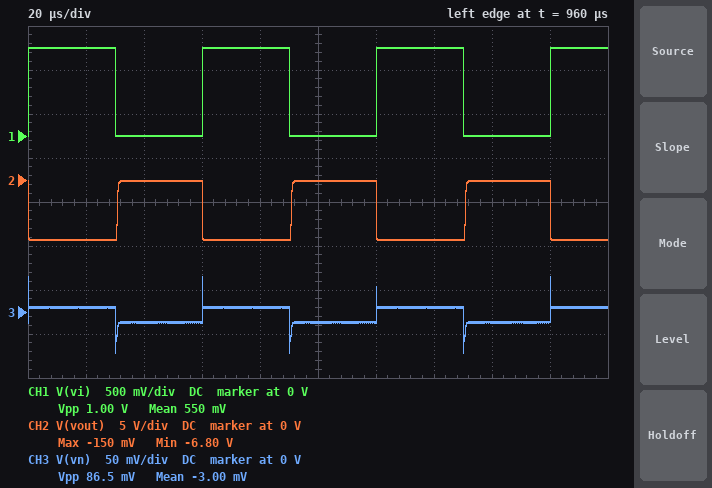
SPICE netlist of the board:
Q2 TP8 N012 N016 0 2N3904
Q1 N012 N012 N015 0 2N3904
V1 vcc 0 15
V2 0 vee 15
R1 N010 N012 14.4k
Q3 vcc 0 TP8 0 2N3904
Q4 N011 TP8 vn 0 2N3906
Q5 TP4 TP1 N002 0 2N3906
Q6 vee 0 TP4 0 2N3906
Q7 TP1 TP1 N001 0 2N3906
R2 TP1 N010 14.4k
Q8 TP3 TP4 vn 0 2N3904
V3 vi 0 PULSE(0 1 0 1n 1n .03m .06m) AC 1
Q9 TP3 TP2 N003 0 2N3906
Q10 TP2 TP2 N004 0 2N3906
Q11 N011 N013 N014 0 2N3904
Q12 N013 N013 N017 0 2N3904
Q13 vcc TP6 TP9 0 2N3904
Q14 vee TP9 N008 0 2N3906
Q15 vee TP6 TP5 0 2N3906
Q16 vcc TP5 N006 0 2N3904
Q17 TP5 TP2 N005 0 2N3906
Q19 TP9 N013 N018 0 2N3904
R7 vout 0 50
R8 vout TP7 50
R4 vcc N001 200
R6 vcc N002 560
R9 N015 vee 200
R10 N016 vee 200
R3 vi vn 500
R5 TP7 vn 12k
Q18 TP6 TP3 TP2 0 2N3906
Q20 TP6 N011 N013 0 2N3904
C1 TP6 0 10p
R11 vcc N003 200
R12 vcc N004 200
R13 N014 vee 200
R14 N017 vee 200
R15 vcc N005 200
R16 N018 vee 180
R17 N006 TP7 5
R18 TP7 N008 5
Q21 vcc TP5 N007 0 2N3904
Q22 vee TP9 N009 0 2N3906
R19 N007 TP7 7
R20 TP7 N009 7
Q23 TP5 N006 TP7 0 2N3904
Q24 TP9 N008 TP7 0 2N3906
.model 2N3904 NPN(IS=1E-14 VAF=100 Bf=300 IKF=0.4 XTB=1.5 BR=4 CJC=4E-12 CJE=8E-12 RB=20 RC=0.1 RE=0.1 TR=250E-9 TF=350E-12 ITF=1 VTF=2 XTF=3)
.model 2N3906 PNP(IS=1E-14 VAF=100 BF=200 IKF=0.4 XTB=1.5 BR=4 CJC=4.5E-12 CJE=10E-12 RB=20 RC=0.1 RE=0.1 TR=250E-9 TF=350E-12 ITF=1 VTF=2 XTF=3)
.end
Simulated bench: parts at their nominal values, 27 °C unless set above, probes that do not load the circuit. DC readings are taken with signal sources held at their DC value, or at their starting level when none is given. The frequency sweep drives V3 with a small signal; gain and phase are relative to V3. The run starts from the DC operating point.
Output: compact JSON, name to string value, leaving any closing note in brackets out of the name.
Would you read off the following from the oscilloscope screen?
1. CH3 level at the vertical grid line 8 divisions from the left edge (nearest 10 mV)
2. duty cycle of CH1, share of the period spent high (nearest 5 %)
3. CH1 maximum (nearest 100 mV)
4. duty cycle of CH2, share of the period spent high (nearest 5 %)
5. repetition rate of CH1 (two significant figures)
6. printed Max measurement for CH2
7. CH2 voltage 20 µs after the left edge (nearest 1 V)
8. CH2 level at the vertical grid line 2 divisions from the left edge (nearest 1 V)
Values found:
{"CH3 level at the vertical grid line 8 divisions from the left edge": "-10 mV", "duty cycle of CH1, share of the period spent high": "50 %", "CH1 maximum": "1.0 V", "duty cycle of CH2, share of the period spent high": "50 %", "repetition rate of CH1": "17 kHz", "printed Max measurement for CH2": "-150 mV", "CH2 voltage 20 µs after the left edge": "-7 V", "CH2 level at the vertical grid line 2 divisions from the left edge": "0 V"}
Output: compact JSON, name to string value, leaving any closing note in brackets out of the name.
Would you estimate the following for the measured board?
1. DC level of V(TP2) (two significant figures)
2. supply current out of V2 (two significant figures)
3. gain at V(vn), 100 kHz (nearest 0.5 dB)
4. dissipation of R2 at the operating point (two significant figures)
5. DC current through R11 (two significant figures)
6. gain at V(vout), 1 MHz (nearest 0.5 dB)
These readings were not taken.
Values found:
{"DC level of V(TP2)": "14 V", "supply current out of V2": "7.9 mA", "gain at V(vn), 100 kHz": "-45.0 dB", "dissipation of R2 at the operating point": "14 mW", "DC current through R11": "610 µA", "gain at V(vout), 1 MHz": "17.0 dB"}
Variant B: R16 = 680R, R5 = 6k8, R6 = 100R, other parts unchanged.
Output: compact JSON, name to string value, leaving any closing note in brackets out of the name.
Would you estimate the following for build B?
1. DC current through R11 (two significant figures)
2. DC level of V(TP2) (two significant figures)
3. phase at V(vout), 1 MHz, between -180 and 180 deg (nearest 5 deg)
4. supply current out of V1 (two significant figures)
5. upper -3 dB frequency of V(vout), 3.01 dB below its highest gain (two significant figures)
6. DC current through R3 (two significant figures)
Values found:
{"DC current through R11": "1.3 mA", "DC level of V(TP2)": "14 V", "phase at V(vout), 1 MHz, between -180 and 180 deg": "140 deg", "supply current out of V1": "11 mA", "upper -3 dB frequency of V(vout), 3.01 dB below its highest gain": "1.3 MHz", "DC current through R3": "16 µA"}
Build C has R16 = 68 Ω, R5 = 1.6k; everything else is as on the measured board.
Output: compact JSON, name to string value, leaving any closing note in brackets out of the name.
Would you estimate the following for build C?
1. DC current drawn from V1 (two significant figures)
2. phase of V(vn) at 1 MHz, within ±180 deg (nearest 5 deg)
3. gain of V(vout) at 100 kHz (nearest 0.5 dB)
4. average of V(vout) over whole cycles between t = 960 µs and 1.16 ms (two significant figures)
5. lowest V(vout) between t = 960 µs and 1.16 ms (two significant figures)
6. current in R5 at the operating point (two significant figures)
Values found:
{"DC current drawn from V1": "7.0 mA", "phase of V(vn) at 1 MHz, within ±180 deg": "80 deg", "gain of V(vout) at 100 kHz": "4.0 dB", "average of V(vout) over whole cycles between t = 960 µs and 1.16 ms": "-830 mV", "lowest V(vout) between t = 960 µs and 1.16 ms": "-1.6 V", "current in R5 at the operating point": "26 µA"}
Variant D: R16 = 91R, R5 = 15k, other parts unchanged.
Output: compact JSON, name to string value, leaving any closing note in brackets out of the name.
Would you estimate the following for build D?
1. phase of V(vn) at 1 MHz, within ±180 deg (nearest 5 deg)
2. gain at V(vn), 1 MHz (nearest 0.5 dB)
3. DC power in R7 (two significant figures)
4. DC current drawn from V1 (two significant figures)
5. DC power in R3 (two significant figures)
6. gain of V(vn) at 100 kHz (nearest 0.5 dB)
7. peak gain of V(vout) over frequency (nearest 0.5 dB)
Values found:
{"phase of V(vn) at 1 MHz, within ±180 deg": "30 deg", "gain at V(vn), 1 MHz": "-29.0 dB", "DC power in R7": "700 µW", "DC current drawn from V1": "5.8 mA", "DC power in R3": "290 nW", "gain of V(vn) at 100 kHz": "-43.0 dB", "peak gain of V(vout) over frequency": "23.5 dB"}
